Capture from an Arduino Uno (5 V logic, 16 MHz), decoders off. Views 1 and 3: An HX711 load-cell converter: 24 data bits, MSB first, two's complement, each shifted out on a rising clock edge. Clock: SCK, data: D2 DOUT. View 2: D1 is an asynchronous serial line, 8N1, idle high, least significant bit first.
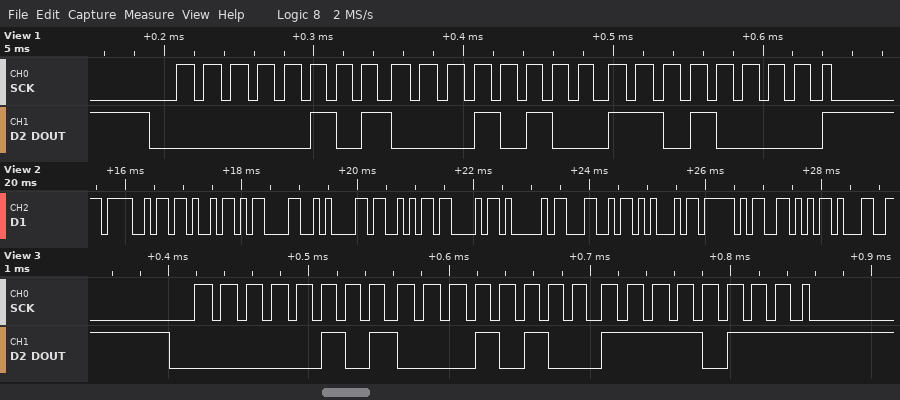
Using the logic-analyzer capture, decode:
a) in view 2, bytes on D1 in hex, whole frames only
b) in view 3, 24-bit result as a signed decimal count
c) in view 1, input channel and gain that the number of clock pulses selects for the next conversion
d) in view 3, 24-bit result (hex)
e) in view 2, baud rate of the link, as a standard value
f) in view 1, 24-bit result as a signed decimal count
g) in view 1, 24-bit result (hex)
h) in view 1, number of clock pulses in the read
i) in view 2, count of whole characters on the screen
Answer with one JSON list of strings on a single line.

["4F 4B 0D 0A 53 43 41 4C 45 5F 56 31", "333047", "channel A, gain 128", "0x0514F7", "9600 baud", "333008", "0x0514D0", "25", "12"]
